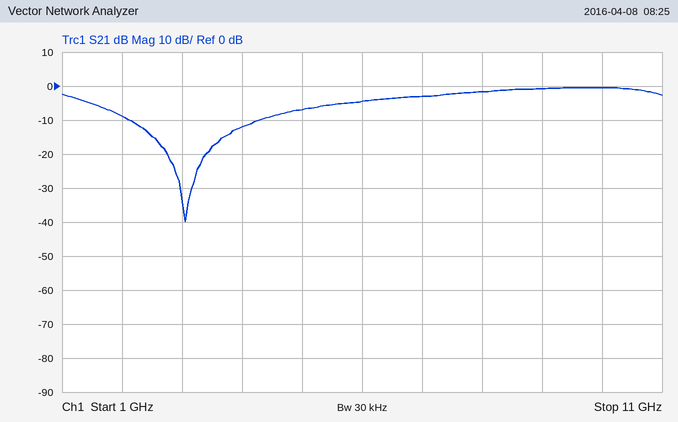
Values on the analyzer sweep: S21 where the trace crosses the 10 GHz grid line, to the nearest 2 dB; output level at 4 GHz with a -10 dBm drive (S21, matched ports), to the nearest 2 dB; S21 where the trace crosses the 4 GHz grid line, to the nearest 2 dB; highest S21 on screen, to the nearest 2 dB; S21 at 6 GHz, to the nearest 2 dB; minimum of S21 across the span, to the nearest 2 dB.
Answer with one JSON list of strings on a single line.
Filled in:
["0 dB", "-22 dBm", "-12 dB", "0 dB", "-4 dB", "-40 dB"]
